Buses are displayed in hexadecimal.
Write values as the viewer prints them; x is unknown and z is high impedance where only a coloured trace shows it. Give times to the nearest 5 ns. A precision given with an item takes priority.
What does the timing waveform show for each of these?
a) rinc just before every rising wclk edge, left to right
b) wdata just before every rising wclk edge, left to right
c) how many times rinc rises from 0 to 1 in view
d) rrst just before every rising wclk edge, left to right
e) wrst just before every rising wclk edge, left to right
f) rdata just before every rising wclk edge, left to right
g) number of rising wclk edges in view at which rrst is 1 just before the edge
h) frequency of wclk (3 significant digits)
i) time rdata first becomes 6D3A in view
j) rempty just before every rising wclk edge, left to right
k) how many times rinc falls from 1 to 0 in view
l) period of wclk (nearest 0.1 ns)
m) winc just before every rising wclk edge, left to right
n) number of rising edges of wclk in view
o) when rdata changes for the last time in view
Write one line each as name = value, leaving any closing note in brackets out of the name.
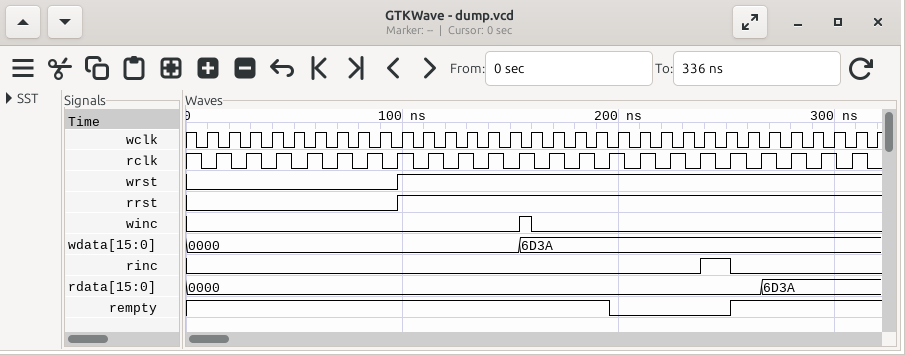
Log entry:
rinc just before every rising wclk edge, left to right = 0 0 0 0 0 0 0 0 0 0 0 0 0 0 0 0 0 0 0 0 0 0 0 1 1 0 0 0 0 0 0 0
wdata just before every rising wclk edge, left to right = 0000, 0000, 0000, 0000, 0000, 0000, 0000, 0000, 0000, 0000, 0000, 0000, 0000, 0000, 0000, 6D3A, 6D3A, 6D3A, 6D3A, 6D3A, 6D3A, 6D3A, 6D3A, 6D3A, 6D3A, 6D3A, 6D3A, 6D3A, 6D3A, 6D3A, 6D3A, 6D3A
how many times rinc rises from 0 to 1 in view = 1
rrst just before every rising wclk edge, left to right = 0 0 0 0 0 0 0 0 0 1 1 1 1 1 1 1 1 1 1 1 1 1 1 1 1 1 1 1 1 1 1 1
wrst just before every rising wclk edge, left to right = 0 0 0 0 0 0 0 0 0 1 1 1 1 1 1 1 1 1 1 1 1 1 1 1 1 1 1 1 1 1 1 1
rdata just before every rising wclk edge, left to right = 0000, 0000, 0000, 0000, 0000, 0000, 0000, 0000, 0000, 0000, 0000, 0000, 0000, 0000, 0000, 0000, 0000, 0000, 0000, 0000, 0000, 0000, 0000, 0000, 0000, 0000, 6D3A, 6D3A, 6D3A, 6D3A, 6D3A, 6D3A
number of rising wclk edges in view at which rrst is 1 just before the edge = 23
frequency of wclk = 100 MHz
time rdata first becomes 6D3A in view = 265 ns
rempty just before every rising wclk edge, left to right = 1 1 1 1 1 1 1 1 1 1 1 1 1 1 1 1 1 1 1 0 0 0 0 0 0 1 1 1 1 1 1 1
how many times rinc falls from 1 to 0 in view = 1
period of wclk = 10 ns
winc just before every rising wclk edge, left to right = 0 0 0 0 0 0 0 0 0 0 0 0 0 0 0 1 0 0 0 0 0 0 0 0 0 0 0 0 0 0 0 0
number of rising edges of wclk in view = 32
when rdata changes for the last time in view = 265 ns
